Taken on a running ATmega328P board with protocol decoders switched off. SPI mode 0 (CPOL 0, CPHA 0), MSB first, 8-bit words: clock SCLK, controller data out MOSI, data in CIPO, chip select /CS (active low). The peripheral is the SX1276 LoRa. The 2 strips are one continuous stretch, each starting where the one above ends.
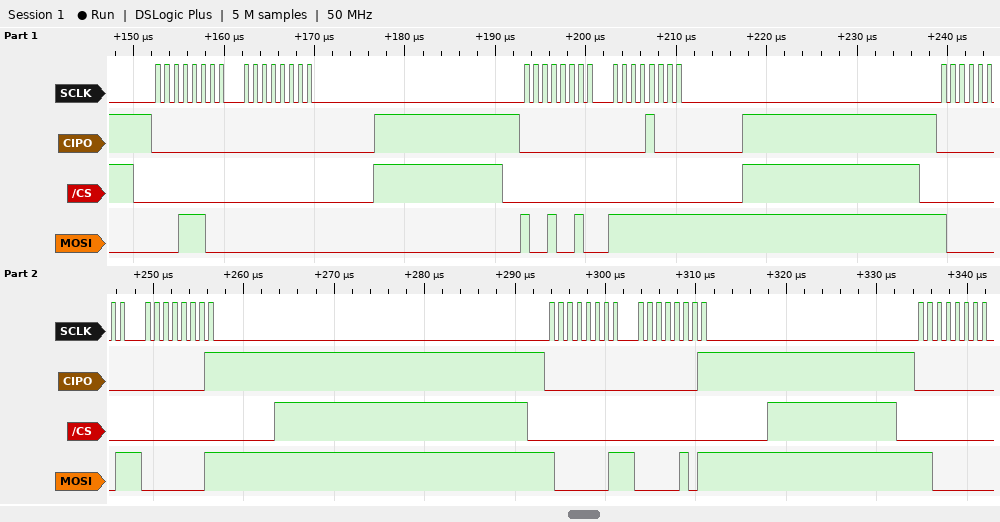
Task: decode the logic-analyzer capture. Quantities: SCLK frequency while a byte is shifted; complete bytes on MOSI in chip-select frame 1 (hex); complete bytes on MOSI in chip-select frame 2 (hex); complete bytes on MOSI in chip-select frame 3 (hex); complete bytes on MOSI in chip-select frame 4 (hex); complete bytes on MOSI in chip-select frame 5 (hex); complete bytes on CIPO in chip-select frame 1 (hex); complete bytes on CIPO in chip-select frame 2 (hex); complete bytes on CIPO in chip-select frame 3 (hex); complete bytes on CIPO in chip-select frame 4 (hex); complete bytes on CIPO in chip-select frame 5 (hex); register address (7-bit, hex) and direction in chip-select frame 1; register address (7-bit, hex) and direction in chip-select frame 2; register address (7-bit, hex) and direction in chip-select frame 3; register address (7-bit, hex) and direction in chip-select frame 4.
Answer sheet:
1 MHz
0x1C 0x00
0x92 0xFF
0x81 0x01
0x81 0x05
0xC0
0x00 0x00
0x00 0x08
0x00 0x01
0x00 0x01
0x00
0x1C read
0x12 write
0x01 write
0x01 write
